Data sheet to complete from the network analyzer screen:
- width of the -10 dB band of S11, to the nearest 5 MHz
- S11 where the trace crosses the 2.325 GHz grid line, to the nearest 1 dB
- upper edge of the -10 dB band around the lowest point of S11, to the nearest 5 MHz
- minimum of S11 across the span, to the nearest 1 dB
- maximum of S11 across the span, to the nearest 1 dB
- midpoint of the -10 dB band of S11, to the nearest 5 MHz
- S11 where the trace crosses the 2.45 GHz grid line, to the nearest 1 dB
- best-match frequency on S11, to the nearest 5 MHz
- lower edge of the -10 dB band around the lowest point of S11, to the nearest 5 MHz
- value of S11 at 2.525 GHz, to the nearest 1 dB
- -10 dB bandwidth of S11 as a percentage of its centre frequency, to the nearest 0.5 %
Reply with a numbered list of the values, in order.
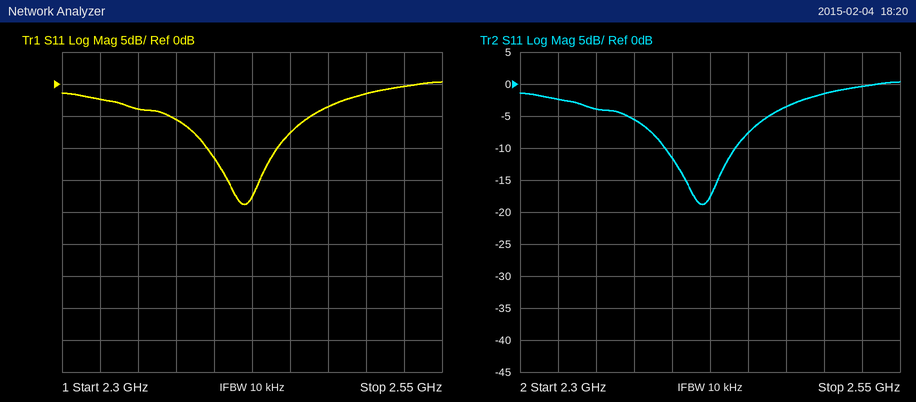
1. 45 MHz
2. -2 dB
3. 2.440 GHz
4. -19 dB
5. 0 dB
6. 2.420 GHz
7. -8 dB
8. 2.420 GHz
9. 2.395 GHz
10. 0 dB
11. 2.0 %
